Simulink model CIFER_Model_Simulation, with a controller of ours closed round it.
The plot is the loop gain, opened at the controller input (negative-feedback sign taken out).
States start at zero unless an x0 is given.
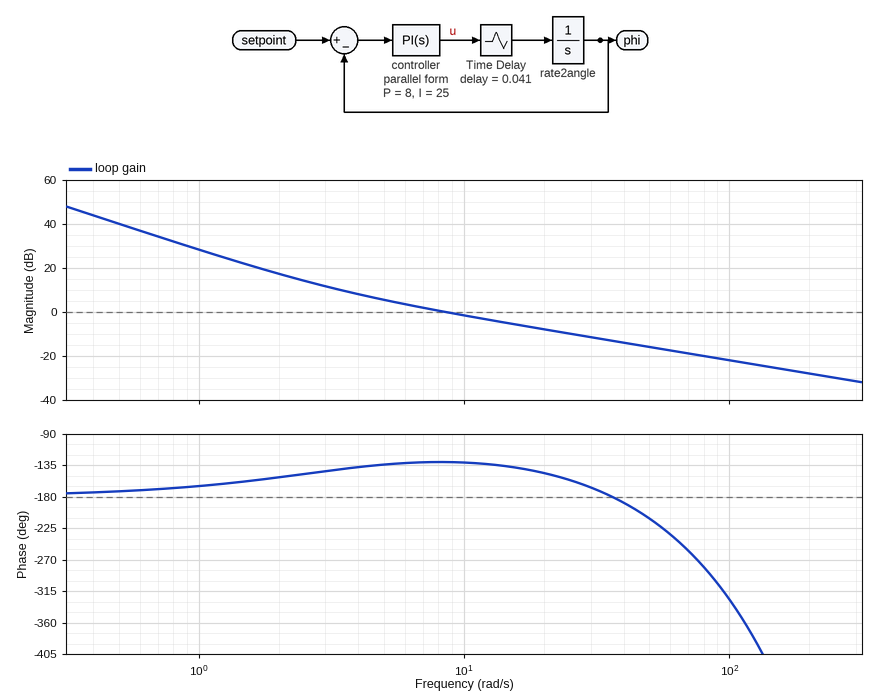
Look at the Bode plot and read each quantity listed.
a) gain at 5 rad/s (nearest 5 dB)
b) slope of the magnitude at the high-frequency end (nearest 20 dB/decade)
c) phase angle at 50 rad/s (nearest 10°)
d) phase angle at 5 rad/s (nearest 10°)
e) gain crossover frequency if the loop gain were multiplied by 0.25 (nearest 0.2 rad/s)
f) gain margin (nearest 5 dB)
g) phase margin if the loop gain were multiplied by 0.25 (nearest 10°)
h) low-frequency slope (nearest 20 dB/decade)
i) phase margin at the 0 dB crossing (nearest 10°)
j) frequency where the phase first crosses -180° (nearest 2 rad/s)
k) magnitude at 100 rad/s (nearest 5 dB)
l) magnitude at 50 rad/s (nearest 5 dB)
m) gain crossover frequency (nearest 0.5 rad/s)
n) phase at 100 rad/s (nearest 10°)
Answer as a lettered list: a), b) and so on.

a) 5 dB
b) -20 dB/decade
c) -210°
d) -130°
e) 3.0 rad/s
f) 15 dB
g) 40°
h) -40 dB/decade
i) 50°
j) 36 rad/s
k) -20 dB
l) -15 dB
m) 8.5 rad/s
n) -330°
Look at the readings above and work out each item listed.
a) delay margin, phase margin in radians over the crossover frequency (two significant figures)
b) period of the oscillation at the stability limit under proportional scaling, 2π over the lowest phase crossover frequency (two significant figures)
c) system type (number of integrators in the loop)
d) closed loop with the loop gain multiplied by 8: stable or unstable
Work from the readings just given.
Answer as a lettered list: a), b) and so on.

a) 0.10 s
b) 0.17 s
c) 2
d) unstable
